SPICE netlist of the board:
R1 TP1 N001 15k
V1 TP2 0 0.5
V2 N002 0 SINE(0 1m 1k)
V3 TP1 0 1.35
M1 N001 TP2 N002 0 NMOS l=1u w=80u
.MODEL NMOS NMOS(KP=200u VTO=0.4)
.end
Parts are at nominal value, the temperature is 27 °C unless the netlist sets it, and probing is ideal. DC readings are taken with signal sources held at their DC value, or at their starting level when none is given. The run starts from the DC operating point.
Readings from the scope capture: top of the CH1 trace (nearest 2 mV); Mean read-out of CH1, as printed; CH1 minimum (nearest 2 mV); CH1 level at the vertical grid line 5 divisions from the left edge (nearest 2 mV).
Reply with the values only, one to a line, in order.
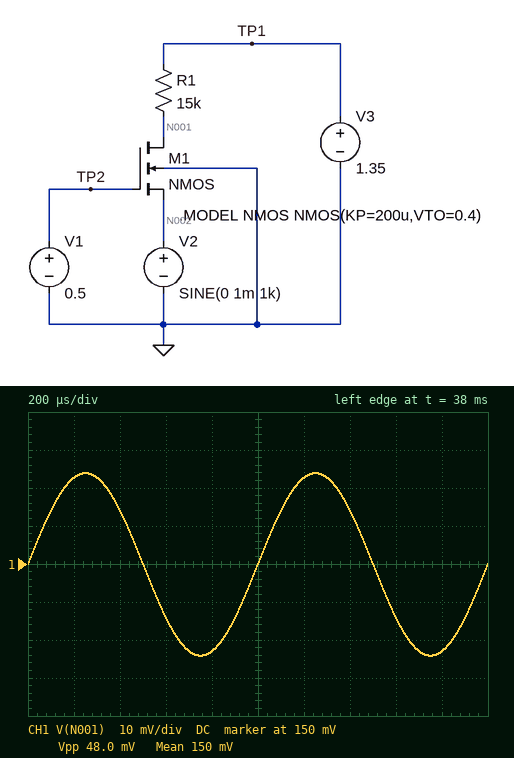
174 mV
150 mV
126 mV
150 mV
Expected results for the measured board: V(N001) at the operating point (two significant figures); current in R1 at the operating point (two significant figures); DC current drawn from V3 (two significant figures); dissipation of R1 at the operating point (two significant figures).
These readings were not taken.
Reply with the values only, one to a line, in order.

150 mV
80 µA
80 µA
96 µW
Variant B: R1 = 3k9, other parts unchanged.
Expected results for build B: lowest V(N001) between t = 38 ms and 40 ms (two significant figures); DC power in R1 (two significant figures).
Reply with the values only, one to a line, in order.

1.0 V
25 µW
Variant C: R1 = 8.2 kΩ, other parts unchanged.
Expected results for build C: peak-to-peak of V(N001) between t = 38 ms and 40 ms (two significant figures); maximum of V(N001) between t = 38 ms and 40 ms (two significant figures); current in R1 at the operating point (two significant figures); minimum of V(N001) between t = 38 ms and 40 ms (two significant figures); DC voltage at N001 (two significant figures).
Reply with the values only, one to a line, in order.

26 mV
710 mV
80 µA
680 mV
690 mV
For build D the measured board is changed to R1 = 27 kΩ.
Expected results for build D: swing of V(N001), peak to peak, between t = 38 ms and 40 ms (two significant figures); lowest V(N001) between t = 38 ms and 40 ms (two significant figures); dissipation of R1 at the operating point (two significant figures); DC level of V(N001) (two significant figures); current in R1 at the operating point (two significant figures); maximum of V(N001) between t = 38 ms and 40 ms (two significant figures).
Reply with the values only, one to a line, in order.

3.1 mV
36 mV
64 µW
37 mV
49 µA
39 mV
